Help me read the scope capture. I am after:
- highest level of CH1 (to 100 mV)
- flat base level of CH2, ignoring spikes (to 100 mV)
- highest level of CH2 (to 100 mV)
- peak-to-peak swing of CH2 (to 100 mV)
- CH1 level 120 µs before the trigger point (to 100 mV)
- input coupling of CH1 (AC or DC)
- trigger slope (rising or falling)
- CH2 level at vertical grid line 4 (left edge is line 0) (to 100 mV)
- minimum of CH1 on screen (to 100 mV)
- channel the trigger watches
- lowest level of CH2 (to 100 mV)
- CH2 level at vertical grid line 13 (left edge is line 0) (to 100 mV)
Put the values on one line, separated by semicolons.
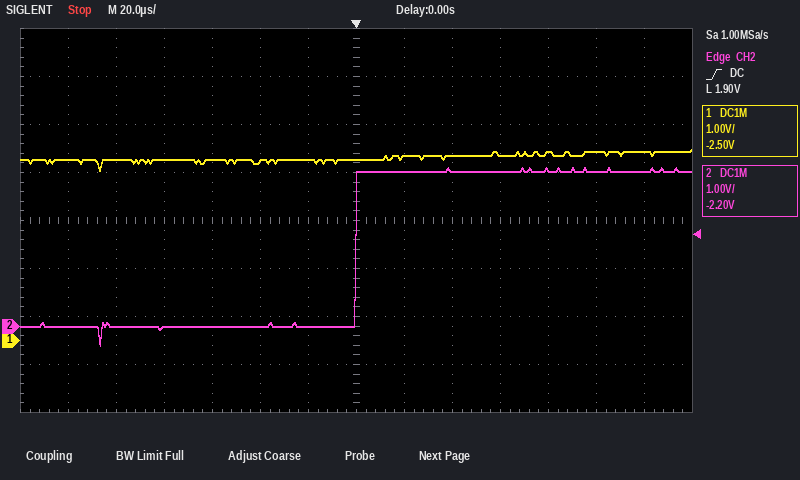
4.0 V; 0.0 V; 3.3 V; 3.7 V; 3.8 V; DC; rising; 0.0 V; 3.5 V; CH2; -400 mV; 3.2 V
